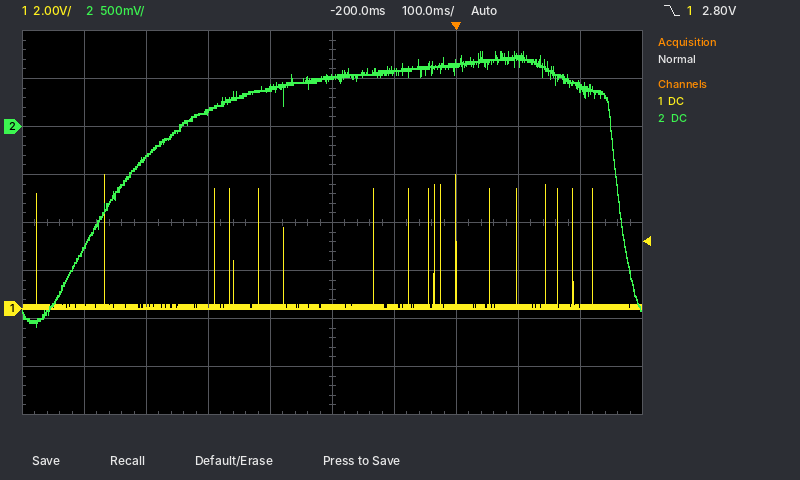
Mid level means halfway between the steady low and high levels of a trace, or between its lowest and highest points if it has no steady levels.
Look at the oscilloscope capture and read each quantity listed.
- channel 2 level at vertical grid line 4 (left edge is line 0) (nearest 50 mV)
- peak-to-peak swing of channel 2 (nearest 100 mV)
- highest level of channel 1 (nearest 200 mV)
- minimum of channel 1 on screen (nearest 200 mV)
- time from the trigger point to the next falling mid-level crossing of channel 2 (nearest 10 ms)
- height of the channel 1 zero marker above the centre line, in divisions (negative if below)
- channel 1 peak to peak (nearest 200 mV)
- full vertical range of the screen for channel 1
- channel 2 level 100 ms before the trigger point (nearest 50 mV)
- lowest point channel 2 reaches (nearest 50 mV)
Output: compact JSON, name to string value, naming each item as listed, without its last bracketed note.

{"channel 2 level at vertical grid line 4 (left edge is line 0)": "400 mV", "peak-to-peak swing of channel 2": "2.90 V", "highest level of channel 1": "5.6 V", "minimum of channel 1 on screen": "0.0 V", "time from the trigger point to the next falling mid-level crossing of channel 2": "260 ms", "height of the channel 1 zero marker above the centre line, in divisions": "-1.8 div", "channel 1 peak to peak": "5.6 V", "full vertical range of the screen for channel 1": "16 V", "channel 2 level 100 ms before the trigger point": "600 mV", "lowest point channel 2 reaches": "-2.10 V"}
